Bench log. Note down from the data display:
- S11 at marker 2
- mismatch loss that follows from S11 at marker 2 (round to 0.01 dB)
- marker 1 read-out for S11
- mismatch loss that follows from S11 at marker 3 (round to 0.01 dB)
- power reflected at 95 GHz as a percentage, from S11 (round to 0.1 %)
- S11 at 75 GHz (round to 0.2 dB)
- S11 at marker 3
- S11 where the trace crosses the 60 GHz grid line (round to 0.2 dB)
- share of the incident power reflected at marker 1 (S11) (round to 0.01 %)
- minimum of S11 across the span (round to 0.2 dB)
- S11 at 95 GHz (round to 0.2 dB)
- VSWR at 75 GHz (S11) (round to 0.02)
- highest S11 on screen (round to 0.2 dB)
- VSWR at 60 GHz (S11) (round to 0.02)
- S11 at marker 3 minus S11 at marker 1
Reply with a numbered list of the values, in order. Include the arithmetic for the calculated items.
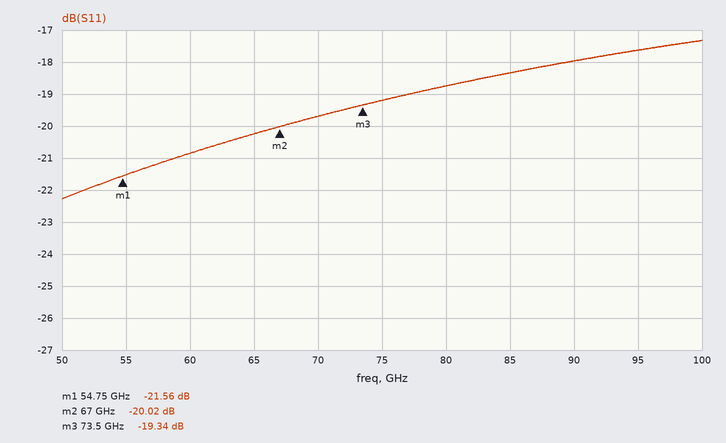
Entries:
1. -20.02 dB
2. −10 log10(1 − 10^(-20.02/10)) ≈ 0.04 dB
3. -21.56 dB
4. −10 log10(1 − 10^(-19.34/10)) ≈ 0.05 dB
5. 10^(-17.6/10) ≈ 1.7 %
6. -19.2 dB
7. -19.34 dB
8. -20.8 dB
9. 10^(-21.56/10) ≈ 0.70 %
10. -22.2 dB
11. -17.6 dB
12. |Γ| = 10^(-19.2/20) = 0.1096; VSWR = (1 + 0.1096)/(1 − 0.1096) ≈ 1.25, so 1.24 to the nearest 0.02
13. -17.4 dB
14. |Γ| = 10^(-20.8/20) = 0.0912; VSWR = (1 + 0.0912)/(1 − 0.0912) ≈ 1.20
15. -19.34 − (-21.56) = 2.22 dB
